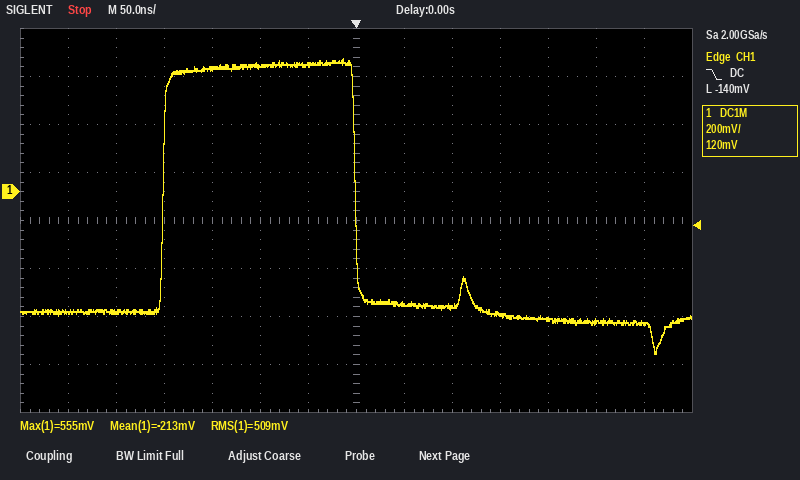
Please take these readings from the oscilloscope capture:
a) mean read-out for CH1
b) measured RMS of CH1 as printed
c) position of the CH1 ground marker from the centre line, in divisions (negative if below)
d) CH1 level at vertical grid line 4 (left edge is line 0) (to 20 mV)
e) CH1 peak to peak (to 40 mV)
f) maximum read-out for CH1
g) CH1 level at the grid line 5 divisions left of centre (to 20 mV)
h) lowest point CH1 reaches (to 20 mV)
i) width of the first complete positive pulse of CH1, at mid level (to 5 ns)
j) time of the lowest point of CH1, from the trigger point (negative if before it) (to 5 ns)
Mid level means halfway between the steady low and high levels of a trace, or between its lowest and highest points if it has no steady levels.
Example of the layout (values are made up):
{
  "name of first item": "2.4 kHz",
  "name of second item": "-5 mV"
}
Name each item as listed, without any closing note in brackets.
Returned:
{
  "mean read-out for CH1": "-213 mV",
  "measured RMS of CH1 as printed": "509 mV",
  "position of the CH1 ground marker from the centre line, in divisions": "+0.6 div",
  "CH1 level at vertical grid line 4 (left edge is line 0)": "520 mV",
  "CH1 peak to peak": "1.24 V",
  "maximum read-out for CH1": "555 mV",
  "CH1 level at the grid line 5 divisions left of centre": "-500 mV",
  "lowest point CH1 reaches": "-680 mV",
  "width of the first complete positive pulse of CH1, at mid level": "200 ns",
  "time of the lowest point of CH1, from the trigger point (negative if before it)": "+310 ns"
}
